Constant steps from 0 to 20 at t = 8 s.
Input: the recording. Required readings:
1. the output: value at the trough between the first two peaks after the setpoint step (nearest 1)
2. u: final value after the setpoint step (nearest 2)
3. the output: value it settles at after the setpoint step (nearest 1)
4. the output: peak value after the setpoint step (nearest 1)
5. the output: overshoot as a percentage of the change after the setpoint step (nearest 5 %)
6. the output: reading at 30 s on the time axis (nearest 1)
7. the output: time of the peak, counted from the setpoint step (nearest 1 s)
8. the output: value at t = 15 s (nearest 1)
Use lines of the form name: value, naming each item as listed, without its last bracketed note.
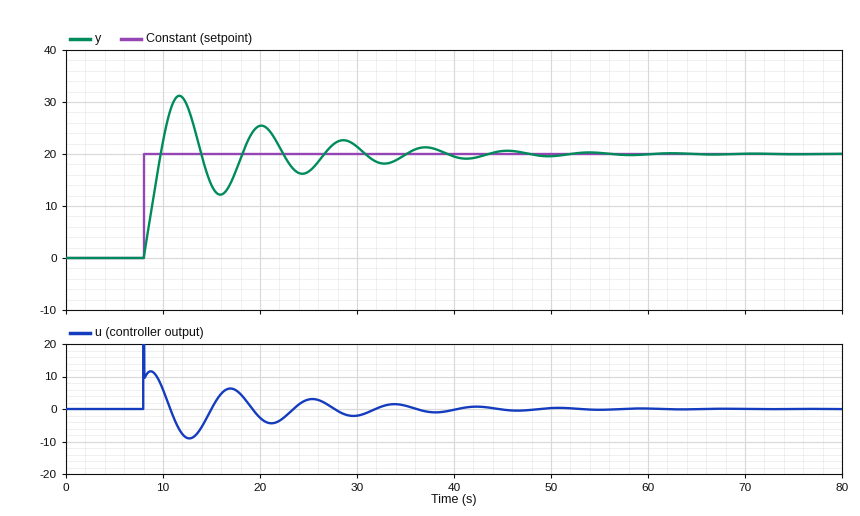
the output: value at the trough between the first two peaks after the setpoint step: 12
u: final value after the setpoint step: 0
the output: value it settles at after the setpoint step: 20
the output: peak value after the setpoint step: 31
the output: overshoot as a percentage of the change after the setpoint step: 55 %
the output: reading at 30 s on the time axis: 21
the output: time of the peak, counted from the setpoint step: 4 s
the output: value at t = 15 s: 14
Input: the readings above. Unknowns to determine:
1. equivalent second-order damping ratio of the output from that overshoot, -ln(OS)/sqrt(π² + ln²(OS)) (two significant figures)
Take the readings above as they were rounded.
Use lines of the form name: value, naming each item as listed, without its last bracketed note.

equivalent second-order damping ratio of the output from that overshoot, -ln(OS)/sqrt(π² + ln²(OS)): 0.19
